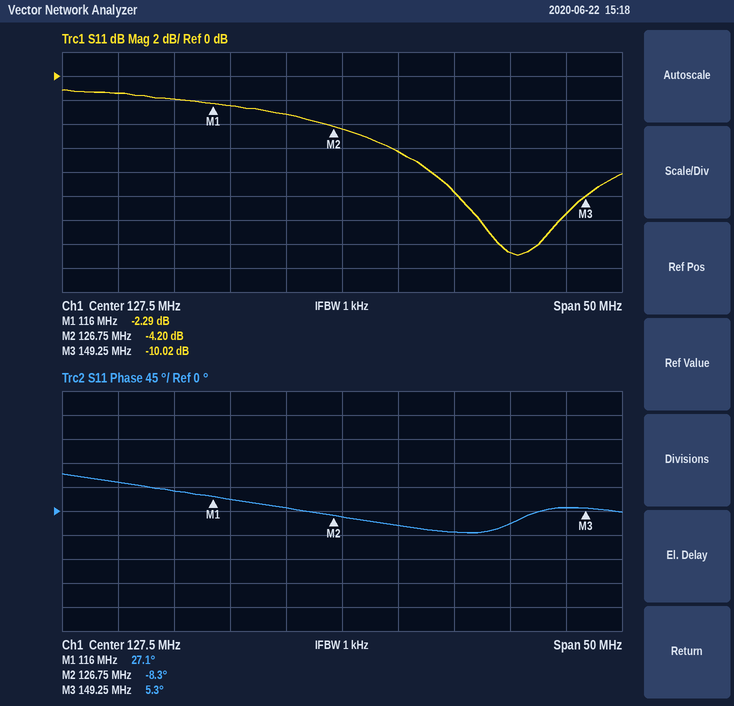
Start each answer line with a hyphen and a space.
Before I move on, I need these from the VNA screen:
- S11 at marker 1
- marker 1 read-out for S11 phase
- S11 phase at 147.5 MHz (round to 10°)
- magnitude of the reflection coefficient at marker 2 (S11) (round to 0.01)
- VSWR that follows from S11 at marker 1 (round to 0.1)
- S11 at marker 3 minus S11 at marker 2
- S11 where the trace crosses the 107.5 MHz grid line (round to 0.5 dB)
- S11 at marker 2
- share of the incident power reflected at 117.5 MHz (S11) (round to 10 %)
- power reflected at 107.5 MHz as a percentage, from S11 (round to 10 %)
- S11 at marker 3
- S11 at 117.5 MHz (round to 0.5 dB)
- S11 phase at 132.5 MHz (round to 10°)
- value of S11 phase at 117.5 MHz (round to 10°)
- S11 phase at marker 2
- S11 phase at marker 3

- -2.29 dB
- 27.1°
- 10°
- 0.62
- 7.6
- -5.82 dB
- -1.5 dB
- -4.20 dB
- 60 %
- 70 %
- -10.02 dB
- -2.5 dB
- -30°
- 20°
- -8.3°
- 5.3°
